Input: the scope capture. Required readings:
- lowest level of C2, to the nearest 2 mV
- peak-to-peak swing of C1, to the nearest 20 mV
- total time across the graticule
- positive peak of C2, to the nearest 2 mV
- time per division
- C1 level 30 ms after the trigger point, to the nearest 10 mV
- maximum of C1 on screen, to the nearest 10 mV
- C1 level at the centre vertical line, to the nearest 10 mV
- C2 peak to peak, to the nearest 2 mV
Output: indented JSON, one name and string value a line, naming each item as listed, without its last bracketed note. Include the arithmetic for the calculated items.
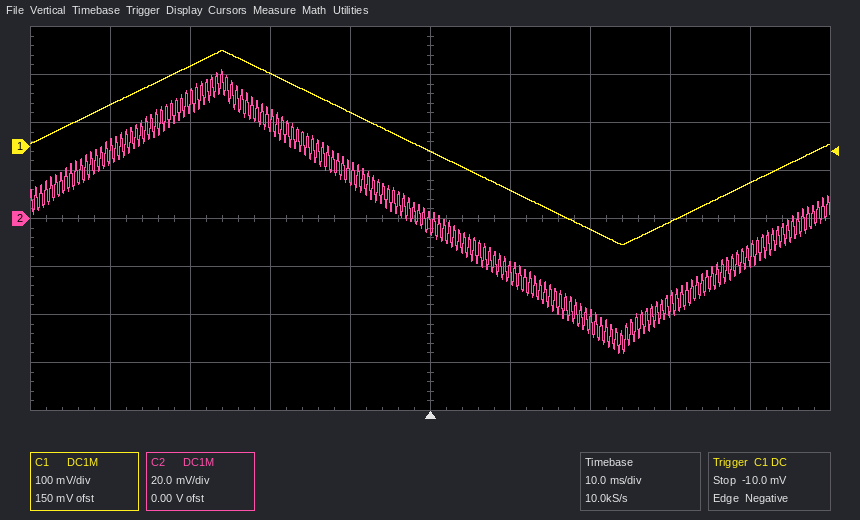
{
  "lowest level of C2, to the nearest 2 mV": "-56 mV",
  "peak-to-peak swing of C1, to the nearest 20 mV": "400 mV",
  "total time across the graticule": "100 ms",
  "positive peak of C2, to the nearest 2 mV": "62 mV",
  "time per division": "10 ms",
  "C1 level 30 ms after the trigger point, to the nearest 10 mV": "-160 mV",
  "maximum of C1 on screen, to the nearest 10 mV": "200 mV",
  "C1 level at the centre vertical line, to the nearest 10 mV": "-10 mV",
  "C2 peak to peak, to the nearest 2 mV": "62 mV − (-56 mV) = 118 mV"
}
